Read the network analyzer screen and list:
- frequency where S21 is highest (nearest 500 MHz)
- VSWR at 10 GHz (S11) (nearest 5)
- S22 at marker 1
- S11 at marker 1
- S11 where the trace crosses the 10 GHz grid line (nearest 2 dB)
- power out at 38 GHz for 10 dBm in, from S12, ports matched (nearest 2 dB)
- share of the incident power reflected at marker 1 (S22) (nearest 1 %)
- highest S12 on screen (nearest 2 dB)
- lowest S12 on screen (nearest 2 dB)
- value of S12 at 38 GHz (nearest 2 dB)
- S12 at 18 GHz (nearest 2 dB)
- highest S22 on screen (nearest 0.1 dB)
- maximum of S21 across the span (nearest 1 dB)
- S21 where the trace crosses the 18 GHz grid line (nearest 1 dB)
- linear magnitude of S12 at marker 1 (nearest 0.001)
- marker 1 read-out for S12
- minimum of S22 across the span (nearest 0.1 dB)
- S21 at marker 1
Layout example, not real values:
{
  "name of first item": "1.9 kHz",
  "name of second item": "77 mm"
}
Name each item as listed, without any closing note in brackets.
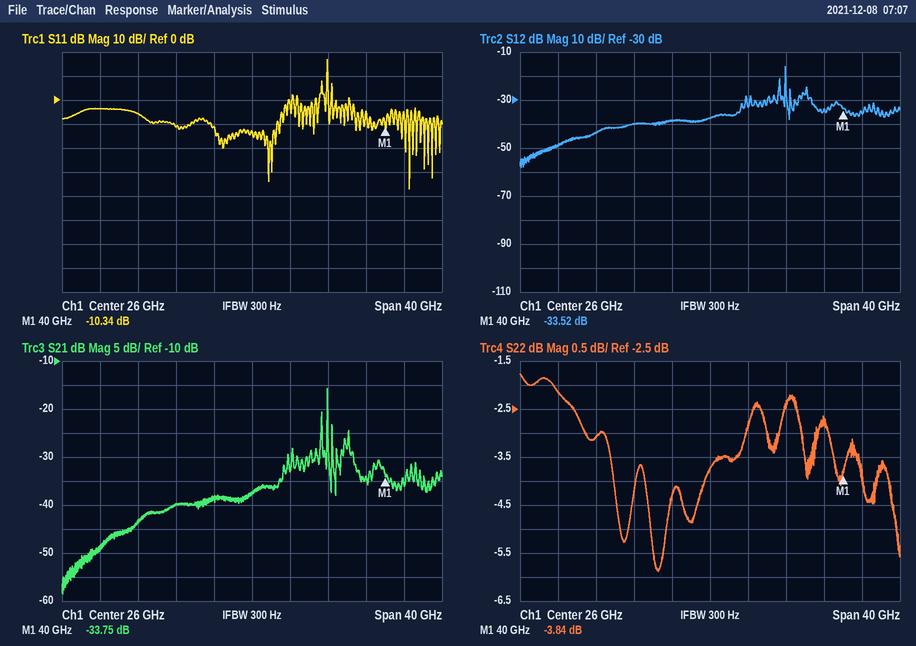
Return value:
{
  "frequency where S21 is highest": "34.0 GHz",
  "VSWR at 10 GHz (S11)": "5",
  "S22 at marker 1": "-3.84 dB",
  "S11 at marker 1": "-10.34 dB",
  "S11 where the trace crosses the 10 GHz grid line": "-4 dB",
  "power out at 38 GHz for 10 dBm in, from S12, ports matched": "-24 dBm",
  "share of the incident power reflected at marker 1 (S22)": "41 %",
  "highest S12 on screen": "-16 dB",
  "lowest S12 on screen": "-58 dB",
  "value of S12 at 38 GHz": "-34 dB",
  "S12 at 18 GHz": "-40 dB",
  "highest S22 on screen": "-1.8 dB",
  "maximum of S21 across the span": "-16 dB",
  "S21 where the trace crosses the 18 GHz grid line": "-40 dB",
  "linear magnitude of S12 at marker 1": "0.021",
  "marker 1 read-out for S12": "-33.52 dB",
  "minimum of S22 across the span": "-5.9 dB",
  "S21 at marker 1": "-33.75 dB"
}
